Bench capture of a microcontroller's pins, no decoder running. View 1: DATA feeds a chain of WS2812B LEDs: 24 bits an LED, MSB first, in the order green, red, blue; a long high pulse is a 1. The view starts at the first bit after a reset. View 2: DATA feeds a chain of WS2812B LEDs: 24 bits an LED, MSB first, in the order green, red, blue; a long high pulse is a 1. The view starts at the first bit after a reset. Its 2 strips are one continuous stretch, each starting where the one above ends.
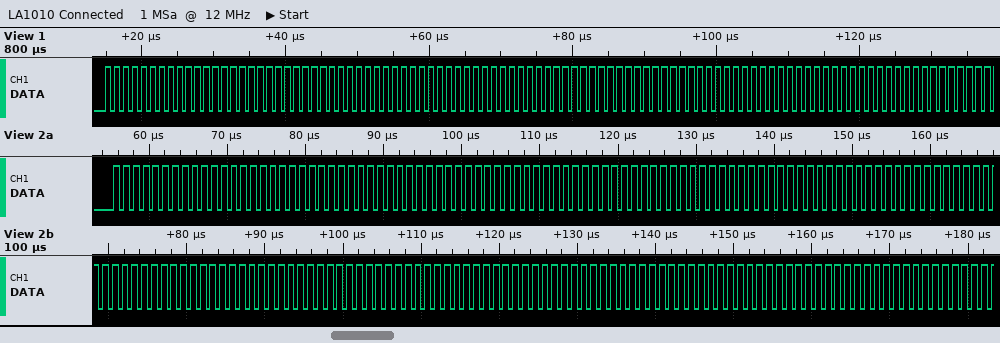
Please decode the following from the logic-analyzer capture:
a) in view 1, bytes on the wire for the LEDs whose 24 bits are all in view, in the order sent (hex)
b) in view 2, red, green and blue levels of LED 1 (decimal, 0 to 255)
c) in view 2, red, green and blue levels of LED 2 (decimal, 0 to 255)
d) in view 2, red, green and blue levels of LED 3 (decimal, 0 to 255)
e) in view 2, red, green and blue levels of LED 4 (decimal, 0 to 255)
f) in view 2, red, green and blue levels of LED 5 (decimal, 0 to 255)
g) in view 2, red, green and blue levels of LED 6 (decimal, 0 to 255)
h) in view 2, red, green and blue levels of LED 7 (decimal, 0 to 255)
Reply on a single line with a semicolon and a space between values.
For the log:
FF FF FF FF FF FF FF FF FF FF FF FF; 255, 255, 255; 255, 255, 255; 255, 255, 255; 255, 255, 255; 255, 255, 255; 255, 255, 255; 255, 255, 255
